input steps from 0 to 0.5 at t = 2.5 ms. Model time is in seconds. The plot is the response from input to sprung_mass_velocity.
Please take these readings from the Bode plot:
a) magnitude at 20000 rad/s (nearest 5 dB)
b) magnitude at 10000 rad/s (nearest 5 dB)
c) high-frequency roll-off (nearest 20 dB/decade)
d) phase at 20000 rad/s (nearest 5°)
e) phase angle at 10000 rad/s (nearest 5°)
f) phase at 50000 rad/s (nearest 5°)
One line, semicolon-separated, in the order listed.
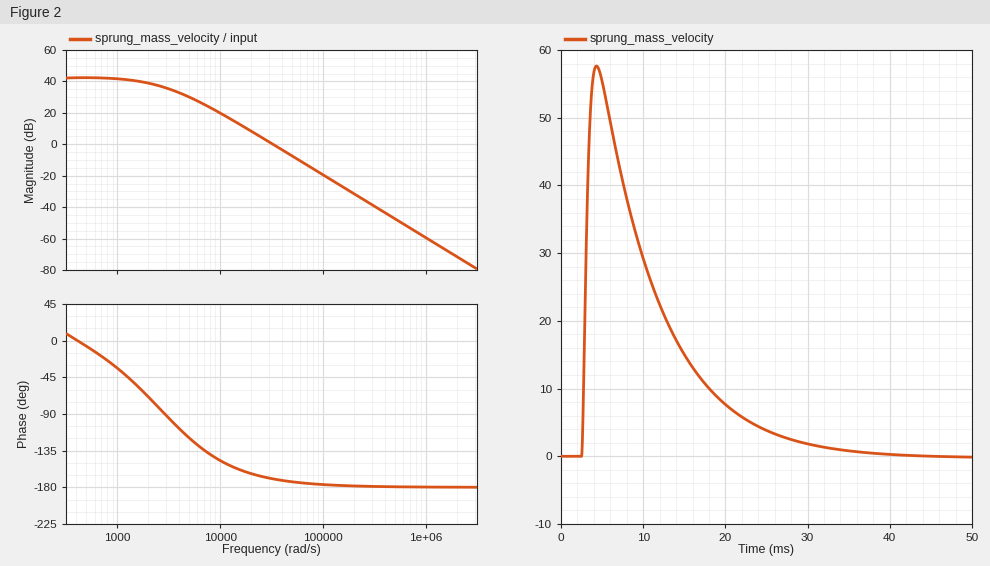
10 dB; 20 dB; -40 dB/decade; -165°; -145°; -175°
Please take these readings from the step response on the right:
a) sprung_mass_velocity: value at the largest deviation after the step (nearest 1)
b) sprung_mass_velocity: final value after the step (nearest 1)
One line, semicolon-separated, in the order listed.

58; 0
